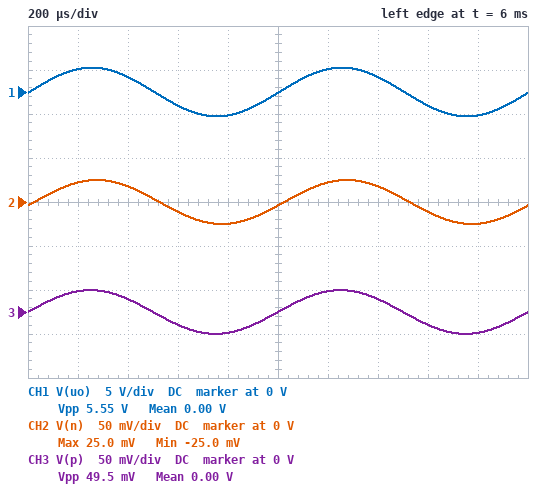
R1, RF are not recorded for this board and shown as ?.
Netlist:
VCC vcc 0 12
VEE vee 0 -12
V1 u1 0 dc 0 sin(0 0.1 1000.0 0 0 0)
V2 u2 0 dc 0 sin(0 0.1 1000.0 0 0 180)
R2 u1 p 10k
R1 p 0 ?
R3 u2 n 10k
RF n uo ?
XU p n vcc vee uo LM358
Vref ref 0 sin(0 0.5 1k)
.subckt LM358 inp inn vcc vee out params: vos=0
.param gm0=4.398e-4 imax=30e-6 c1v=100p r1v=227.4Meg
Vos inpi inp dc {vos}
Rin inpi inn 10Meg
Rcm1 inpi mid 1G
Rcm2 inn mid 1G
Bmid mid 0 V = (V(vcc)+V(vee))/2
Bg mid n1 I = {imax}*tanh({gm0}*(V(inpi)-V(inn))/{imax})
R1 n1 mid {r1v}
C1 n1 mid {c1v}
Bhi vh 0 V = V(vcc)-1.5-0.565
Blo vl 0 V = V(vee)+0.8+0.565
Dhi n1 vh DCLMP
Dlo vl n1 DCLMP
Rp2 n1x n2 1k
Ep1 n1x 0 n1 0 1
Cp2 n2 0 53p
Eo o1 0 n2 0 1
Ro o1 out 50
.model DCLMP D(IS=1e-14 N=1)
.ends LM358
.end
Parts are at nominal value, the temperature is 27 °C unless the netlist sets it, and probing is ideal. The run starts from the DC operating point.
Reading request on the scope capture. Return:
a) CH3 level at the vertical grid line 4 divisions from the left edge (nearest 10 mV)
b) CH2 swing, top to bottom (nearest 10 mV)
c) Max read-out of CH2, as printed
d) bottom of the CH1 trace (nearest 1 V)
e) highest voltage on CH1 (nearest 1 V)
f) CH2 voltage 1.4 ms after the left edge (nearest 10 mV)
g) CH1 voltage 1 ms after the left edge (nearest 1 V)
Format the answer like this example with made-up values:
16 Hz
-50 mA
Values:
-20 mV
50 mV
25.0 mV
-3 V
3 V
20 mV
0 V
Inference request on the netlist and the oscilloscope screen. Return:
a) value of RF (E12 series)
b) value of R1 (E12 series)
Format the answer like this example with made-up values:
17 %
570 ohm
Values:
220 kΩ
3.3 kΩ
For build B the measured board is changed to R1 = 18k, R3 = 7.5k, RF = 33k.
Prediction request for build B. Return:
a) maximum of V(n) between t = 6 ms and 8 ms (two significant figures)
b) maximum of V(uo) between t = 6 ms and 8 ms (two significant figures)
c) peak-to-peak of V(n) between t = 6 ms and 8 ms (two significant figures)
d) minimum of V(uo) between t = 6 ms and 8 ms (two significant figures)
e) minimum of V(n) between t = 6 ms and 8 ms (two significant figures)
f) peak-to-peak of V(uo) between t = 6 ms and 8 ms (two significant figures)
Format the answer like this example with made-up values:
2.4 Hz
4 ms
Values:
64 mV
790 mV
130 mV
-790 mV
-64 mV
1.6 V
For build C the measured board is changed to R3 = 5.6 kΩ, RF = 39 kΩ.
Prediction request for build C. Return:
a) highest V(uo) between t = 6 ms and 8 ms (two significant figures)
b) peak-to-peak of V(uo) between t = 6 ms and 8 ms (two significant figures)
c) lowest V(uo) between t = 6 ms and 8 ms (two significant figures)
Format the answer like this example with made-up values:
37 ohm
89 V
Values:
890 mV
1.8 V
-890 mV
